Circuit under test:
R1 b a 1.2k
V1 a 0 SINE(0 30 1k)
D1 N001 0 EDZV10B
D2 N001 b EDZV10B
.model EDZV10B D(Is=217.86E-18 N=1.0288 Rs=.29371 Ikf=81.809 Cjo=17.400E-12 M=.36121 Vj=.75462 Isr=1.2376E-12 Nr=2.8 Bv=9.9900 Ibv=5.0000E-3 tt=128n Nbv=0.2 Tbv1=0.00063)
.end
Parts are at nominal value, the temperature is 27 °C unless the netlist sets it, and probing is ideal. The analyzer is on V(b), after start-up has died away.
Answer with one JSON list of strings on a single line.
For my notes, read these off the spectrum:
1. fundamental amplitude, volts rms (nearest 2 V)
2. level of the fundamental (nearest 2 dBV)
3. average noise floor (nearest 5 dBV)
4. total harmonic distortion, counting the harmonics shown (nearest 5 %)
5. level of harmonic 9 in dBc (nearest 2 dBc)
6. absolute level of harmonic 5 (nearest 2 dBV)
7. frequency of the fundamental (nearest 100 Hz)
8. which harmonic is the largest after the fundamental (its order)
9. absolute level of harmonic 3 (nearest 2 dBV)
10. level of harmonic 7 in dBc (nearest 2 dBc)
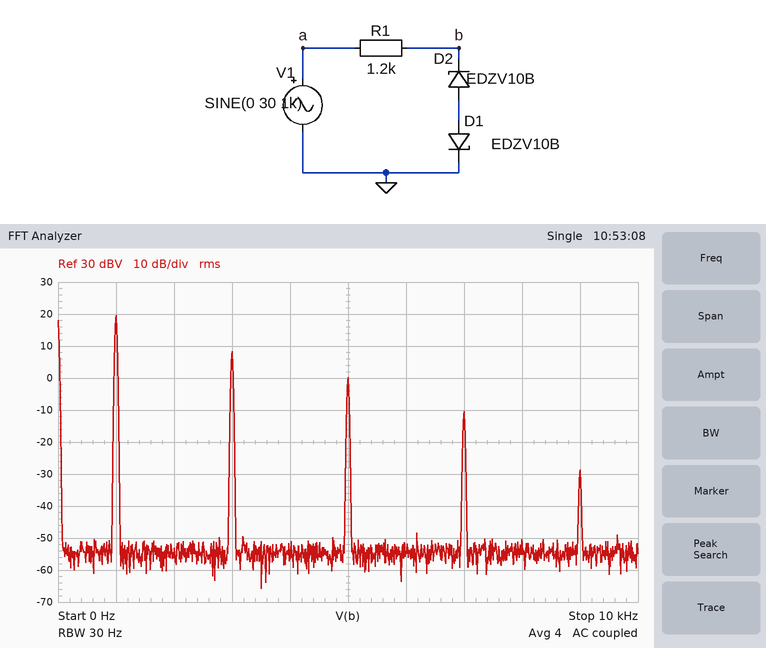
["10 V", "20 dBV", "-55 dBV", "30 %", "-48 dBc", "0 dBV", "1.0 kHz", "3", "8 dBV", "-30 dBc"]
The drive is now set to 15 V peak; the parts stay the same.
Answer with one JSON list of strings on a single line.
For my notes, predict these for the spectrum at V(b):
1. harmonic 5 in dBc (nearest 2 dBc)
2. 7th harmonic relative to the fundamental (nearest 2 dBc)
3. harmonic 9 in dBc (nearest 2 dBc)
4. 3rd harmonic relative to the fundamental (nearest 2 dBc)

["-32 dBc", "-36 dBc", "-40 dBc", "-18 dBc"]
